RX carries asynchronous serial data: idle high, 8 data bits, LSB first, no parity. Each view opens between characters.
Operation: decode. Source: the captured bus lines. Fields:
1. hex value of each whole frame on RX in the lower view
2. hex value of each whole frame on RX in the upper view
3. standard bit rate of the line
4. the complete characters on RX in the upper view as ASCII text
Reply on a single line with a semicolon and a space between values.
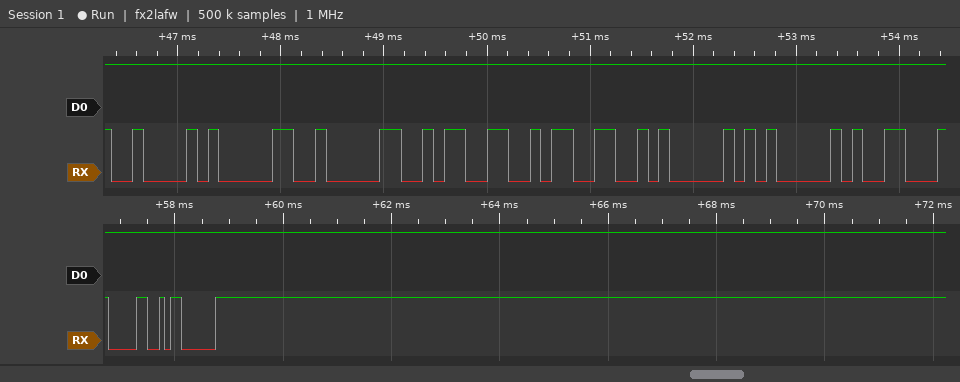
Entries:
30, 03; 42, 30, 30, 33, 33, 41, 41; 9600 baud; "B0033AA"
